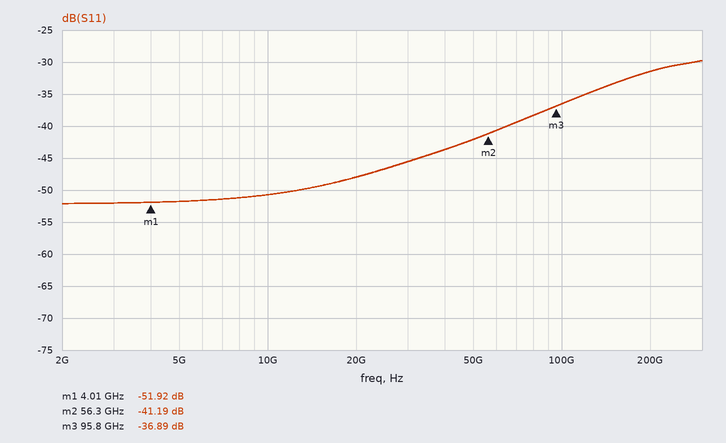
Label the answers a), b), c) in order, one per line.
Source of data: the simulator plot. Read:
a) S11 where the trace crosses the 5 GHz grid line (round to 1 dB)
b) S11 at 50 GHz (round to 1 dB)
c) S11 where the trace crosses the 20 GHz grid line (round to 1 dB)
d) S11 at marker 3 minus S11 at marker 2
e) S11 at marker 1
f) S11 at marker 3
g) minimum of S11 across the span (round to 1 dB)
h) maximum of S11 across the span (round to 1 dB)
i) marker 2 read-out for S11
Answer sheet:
a) -52 dB
b) -42 dB
c) -48 dB
d) 4.30 dB
e) -51.92 dB
f) -36.89 dB
g) -52 dB
h) -30 dB
i) -41.19 dB
